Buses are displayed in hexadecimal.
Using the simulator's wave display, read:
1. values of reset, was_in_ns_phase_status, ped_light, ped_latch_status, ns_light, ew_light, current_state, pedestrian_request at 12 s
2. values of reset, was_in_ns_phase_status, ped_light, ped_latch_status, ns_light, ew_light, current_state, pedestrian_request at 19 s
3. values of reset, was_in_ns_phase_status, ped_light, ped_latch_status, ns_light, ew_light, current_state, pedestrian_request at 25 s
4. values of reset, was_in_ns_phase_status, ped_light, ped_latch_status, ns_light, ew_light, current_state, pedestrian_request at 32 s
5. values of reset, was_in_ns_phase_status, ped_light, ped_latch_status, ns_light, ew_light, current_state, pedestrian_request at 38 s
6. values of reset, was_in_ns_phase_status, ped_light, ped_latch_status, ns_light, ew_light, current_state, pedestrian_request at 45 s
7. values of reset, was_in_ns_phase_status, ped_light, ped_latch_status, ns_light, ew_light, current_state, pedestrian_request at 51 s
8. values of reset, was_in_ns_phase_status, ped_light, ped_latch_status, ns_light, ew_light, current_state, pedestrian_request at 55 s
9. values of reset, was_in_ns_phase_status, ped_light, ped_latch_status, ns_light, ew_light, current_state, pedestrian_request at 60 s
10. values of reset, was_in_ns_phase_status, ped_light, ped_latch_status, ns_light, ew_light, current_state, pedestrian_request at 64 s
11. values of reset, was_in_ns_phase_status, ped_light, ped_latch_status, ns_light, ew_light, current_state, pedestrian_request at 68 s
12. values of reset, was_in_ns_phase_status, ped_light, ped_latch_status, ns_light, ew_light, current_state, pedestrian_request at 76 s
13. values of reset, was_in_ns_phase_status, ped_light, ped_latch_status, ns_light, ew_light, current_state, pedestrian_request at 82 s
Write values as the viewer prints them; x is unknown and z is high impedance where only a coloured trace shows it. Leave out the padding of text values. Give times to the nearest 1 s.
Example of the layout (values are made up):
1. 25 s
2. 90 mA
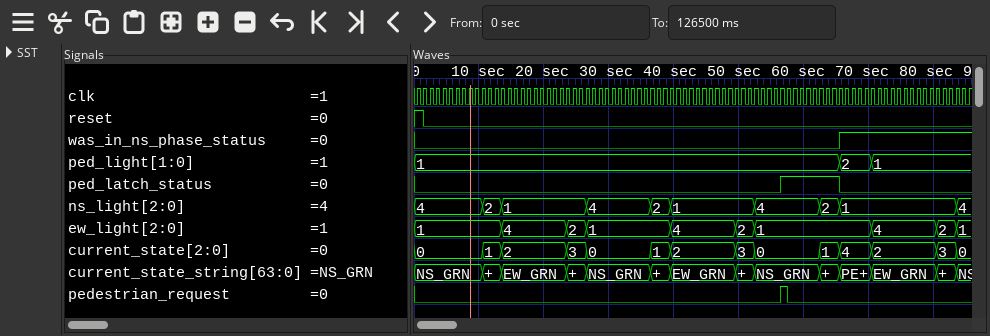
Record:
1. reset=0, was_in_ns_phase_status=0, ped_light=1, ped_latch_status=0, ns_light=2, ew_light=1, current_state=1, pedestrian_request=0
2. reset=0, was_in_ns_phase_status=0, ped_light=1, ped_latch_status=0, ns_light=1, ew_light=4, current_state=2, pedestrian_request=0
3. reset=0, was_in_ns_phase_status=0, ped_light=1, ped_latch_status=0, ns_light=1, ew_light=2, current_state=3, pedestrian_request=0
4. reset=0, was_in_ns_phase_status=0, ped_light=1, ped_latch_status=0, ns_light=4, ew_light=1, current_state=0, pedestrian_request=0
5. reset=0, was_in_ns_phase_status=0, ped_light=1, ped_latch_status=0, ns_light=2, ew_light=1, current_state=1, pedestrian_request=0
6. reset=0, was_in_ns_phase_status=0, ped_light=1, ped_latch_status=0, ns_light=1, ew_light=4, current_state=2, pedestrian_request=0
7. reset=0, was_in_ns_phase_status=0, ped_light=1, ped_latch_status=0, ns_light=1, ew_light=2, current_state=3, pedestrian_request=0
8. reset=0, was_in_ns_phase_status=0, ped_light=1, ped_latch_status=0, ns_light=4, ew_light=1, current_state=0, pedestrian_request=0
9. reset=0, was_in_ns_phase_status=0, ped_light=1, ped_latch_status=1, ns_light=4, ew_light=1, current_state=0, pedestrian_request=0
10. reset=0, was_in_ns_phase_status=0, ped_light=1, ped_latch_status=1, ns_light=2, ew_light=1, current_state=1, pedestrian_request=0
11. reset=0, was_in_ns_phase_status=1, ped_light=2, ped_latch_status=0, ns_light=1, ew_light=1, current_state=4, pedestrian_request=0
12. reset=0, was_in_ns_phase_status=1, ped_light=1, ped_latch_status=0, ns_light=1, ew_light=4, current_state=2, pedestrian_request=0
13. reset=0, was_in_ns_phase_status=1, ped_light=1, ped_latch_status=0, ns_light=1, ew_light=2, current_state=3, pedestrian_request=0
